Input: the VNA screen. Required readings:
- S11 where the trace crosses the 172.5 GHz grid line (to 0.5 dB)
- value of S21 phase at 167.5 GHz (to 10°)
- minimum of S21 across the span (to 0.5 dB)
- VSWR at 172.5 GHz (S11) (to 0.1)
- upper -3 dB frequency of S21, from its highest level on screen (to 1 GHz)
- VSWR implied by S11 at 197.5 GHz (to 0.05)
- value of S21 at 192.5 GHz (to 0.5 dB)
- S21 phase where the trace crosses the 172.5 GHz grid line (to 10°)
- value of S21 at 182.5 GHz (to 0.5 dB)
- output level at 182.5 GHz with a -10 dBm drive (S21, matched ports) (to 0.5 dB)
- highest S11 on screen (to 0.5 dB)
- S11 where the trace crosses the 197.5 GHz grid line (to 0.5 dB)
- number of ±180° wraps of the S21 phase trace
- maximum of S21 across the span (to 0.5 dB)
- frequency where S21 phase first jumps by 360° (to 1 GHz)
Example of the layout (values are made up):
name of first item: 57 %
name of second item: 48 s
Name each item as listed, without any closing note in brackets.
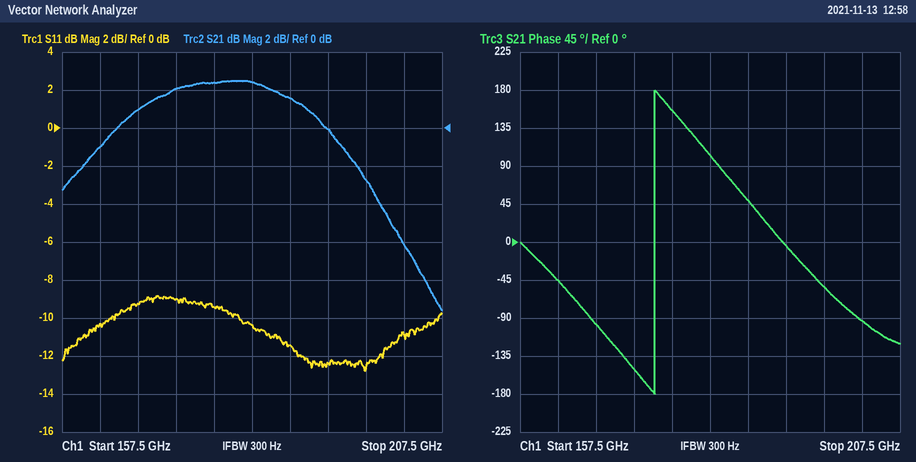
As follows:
S11 where the trace crosses the 172.5 GHz grid line: -9.0 dB
value of S21 phase at 167.5 GHz: -100°
minimum of S21 across the span: -9.5 dB
VSWR at 172.5 GHz (S11): 2.1
upper -3 dB frequency of S21, from its highest level on screen: 193 GHz
VSWR implied by S11 at 197.5 GHz: 1.60
value of S21 at 192.5 GHz: 0.0 dB
S21 phase where the trace crosses the 172.5 GHz grid line: -150°
value of S21 at 182.5 GHz: 2.5 dB
output level at 182.5 GHz with a -10 dBm drive (S21, matched ports): -7.5 dBm
highest S11 on screen: -9.0 dB
S11 where the trace crosses the 197.5 GHz grid line: -12.5 dB
number of ±180° wraps of the S21 phase trace: 1
maximum of S21 across the span: 2.5 dB
frequency where S21 phase first jumps by 360°: 175 GHz
